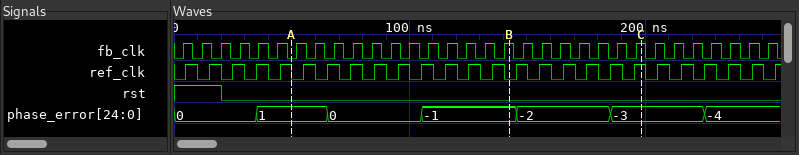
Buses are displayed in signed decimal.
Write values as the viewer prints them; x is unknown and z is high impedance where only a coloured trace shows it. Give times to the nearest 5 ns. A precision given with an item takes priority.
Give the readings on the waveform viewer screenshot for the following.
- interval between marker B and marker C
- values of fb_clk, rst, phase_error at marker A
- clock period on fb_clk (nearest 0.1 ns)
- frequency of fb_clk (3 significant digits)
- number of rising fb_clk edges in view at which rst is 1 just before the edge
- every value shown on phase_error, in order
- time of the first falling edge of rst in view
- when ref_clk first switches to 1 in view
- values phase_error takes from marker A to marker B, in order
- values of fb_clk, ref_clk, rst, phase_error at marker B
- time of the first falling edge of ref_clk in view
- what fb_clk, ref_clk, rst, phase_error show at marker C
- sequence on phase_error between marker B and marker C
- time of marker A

55 ns
fb_clk=0, rst=0, phase_error=1
8 ns
125 MHz
3
0, 1, 0, -1, -2, -3, -4
20 ns
5 ns
1, 0, -1
fb_clk=1, ref_clk=0, rst=0, phase_error=-1
10 ns
fb_clk=1, ref_clk=1, rst=0, phase_error=-3
-1, -2, -3
50 ns
